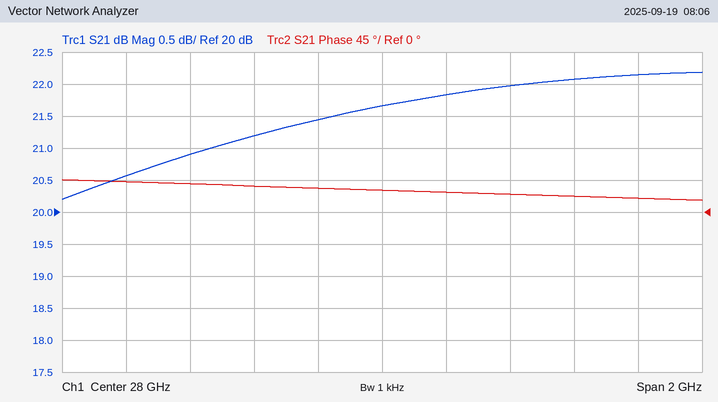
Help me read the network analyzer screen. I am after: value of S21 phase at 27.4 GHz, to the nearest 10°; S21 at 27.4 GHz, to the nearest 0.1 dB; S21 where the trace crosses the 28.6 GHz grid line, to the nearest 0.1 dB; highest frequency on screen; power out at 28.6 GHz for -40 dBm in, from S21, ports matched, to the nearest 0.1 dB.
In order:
40°
20.9 dB
22.1 dB
29 GHz
-17.9 dBm
